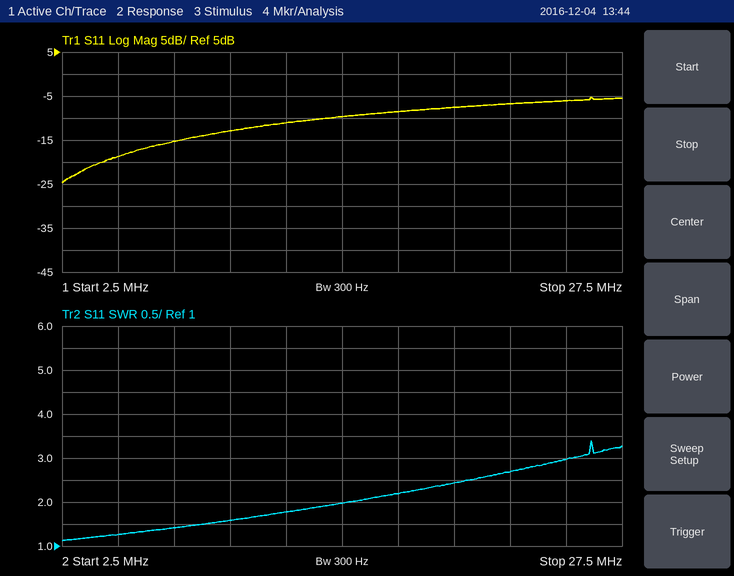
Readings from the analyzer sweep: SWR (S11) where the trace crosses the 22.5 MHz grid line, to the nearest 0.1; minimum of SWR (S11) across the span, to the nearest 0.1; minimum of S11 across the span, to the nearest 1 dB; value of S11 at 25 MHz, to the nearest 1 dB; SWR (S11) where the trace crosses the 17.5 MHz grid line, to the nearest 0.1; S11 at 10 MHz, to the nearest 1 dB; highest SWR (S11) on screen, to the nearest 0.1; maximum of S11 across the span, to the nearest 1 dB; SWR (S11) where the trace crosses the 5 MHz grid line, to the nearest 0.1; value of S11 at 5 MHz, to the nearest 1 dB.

2.7
1.1
-25 dB
-6 dB
2.2
-13 dB
3.4
-5 dB
1.3
-19 dB
